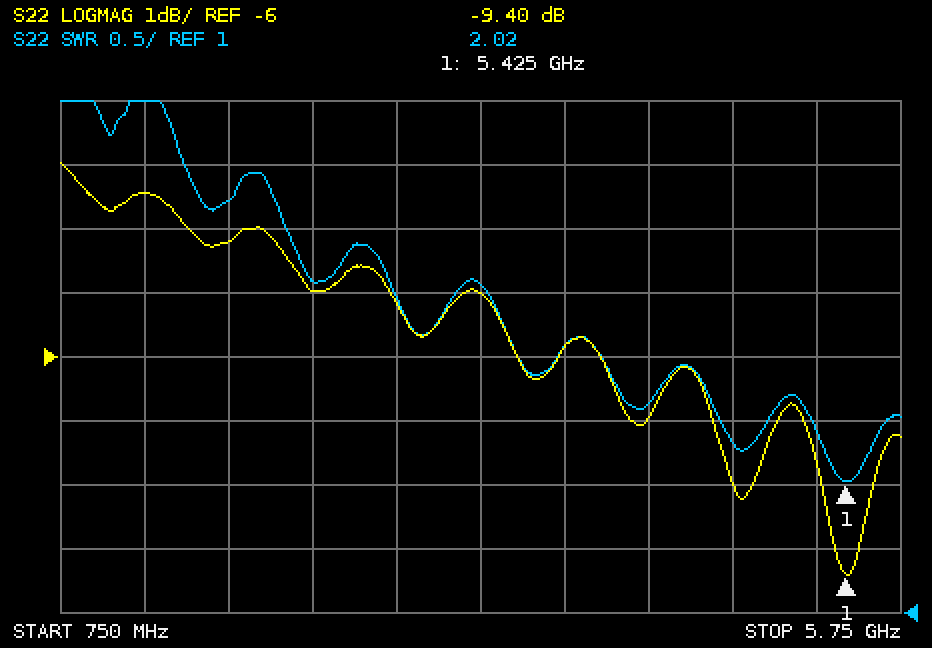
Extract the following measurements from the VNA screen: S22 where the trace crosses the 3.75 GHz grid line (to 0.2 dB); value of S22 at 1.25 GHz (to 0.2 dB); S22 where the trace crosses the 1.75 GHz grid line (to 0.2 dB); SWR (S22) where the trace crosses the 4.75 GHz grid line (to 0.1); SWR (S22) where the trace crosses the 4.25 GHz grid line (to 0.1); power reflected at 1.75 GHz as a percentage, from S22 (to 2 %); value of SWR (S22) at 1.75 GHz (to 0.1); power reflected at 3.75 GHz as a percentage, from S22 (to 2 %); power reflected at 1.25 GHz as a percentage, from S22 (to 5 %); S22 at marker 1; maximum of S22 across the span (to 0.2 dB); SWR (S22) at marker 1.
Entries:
-5.8 dB
-3.4 dB
-4.2 dB
2.3
2.6
38 %
4.2
26 %
45 %
-9.40 dB
-3.0 dB
2.02
